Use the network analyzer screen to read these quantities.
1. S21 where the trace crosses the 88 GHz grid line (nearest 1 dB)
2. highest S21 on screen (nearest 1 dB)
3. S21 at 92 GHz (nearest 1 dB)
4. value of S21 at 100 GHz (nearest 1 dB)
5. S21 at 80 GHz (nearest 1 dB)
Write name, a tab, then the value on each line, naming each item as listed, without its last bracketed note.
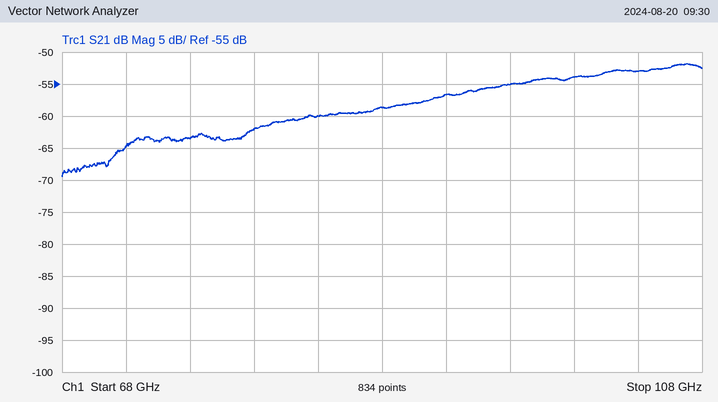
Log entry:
S21 where the trace crosses the 88 GHz grid line	-59 dB
highest S21 on screen	-52 dB
S21 at 92 GHz	-57 dB
value of S21 at 100 GHz	-54 dB
S21 at 80 GHz	-62 dB
